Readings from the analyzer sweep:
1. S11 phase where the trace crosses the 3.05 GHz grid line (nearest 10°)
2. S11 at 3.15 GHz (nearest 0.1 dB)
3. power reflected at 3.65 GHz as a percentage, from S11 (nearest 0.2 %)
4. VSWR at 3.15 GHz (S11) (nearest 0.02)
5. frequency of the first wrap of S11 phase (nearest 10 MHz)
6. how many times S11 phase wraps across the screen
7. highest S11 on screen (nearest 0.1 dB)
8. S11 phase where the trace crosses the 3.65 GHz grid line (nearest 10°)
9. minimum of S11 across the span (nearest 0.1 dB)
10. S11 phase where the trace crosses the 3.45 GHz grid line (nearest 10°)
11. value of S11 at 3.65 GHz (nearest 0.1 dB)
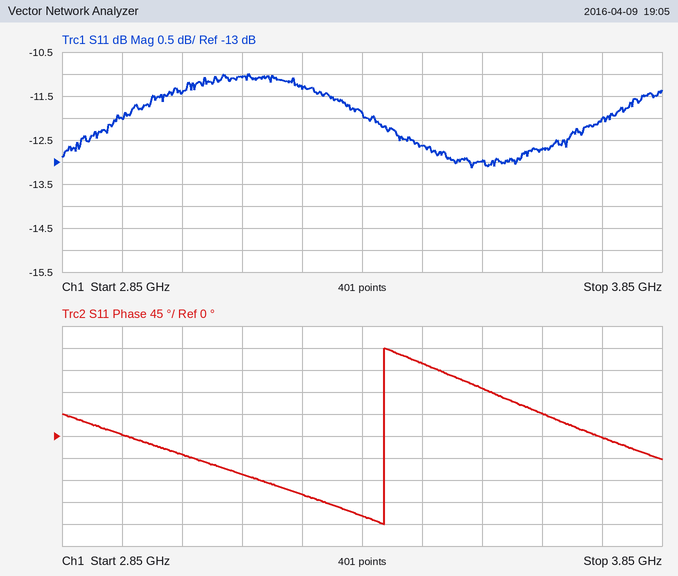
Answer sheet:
-40°
-11.1 dB
5.4 %
1.78
3.39 GHz
1
-11.0 dB
50°
-13.1 dB
150°
-12.7 dB
